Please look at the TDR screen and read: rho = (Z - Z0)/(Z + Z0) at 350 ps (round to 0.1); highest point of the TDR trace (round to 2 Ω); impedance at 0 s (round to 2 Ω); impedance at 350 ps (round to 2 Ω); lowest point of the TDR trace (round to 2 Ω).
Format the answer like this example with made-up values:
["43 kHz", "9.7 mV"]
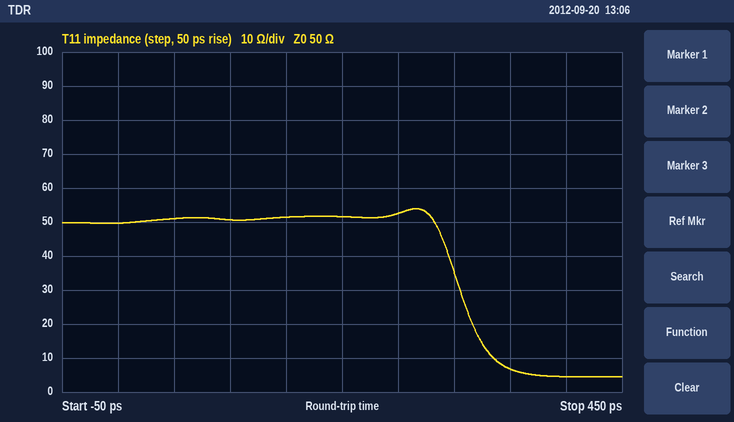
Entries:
["-0.8", "54 Ω", "50 Ω", "6 Ω", "4 Ω"]
